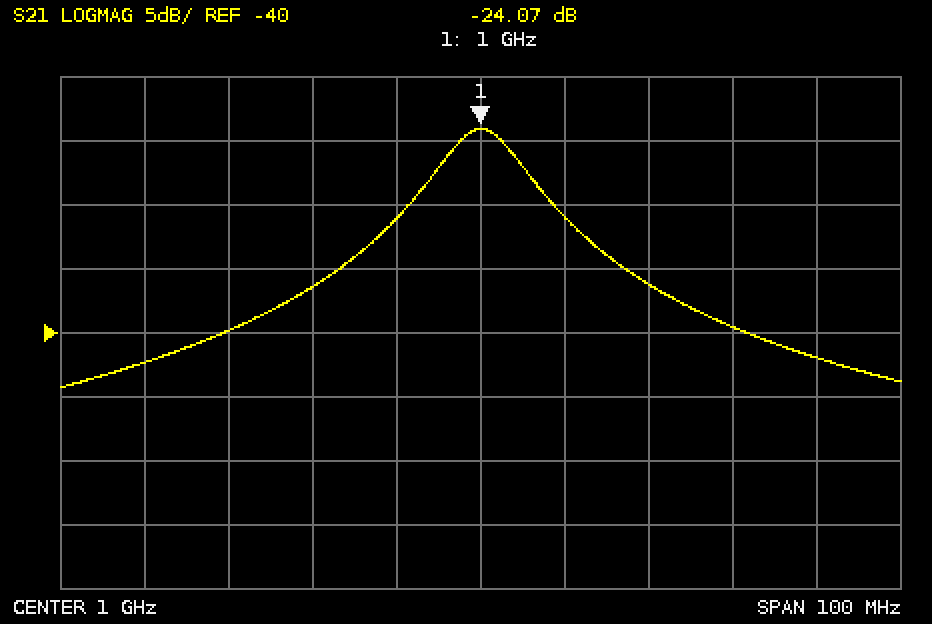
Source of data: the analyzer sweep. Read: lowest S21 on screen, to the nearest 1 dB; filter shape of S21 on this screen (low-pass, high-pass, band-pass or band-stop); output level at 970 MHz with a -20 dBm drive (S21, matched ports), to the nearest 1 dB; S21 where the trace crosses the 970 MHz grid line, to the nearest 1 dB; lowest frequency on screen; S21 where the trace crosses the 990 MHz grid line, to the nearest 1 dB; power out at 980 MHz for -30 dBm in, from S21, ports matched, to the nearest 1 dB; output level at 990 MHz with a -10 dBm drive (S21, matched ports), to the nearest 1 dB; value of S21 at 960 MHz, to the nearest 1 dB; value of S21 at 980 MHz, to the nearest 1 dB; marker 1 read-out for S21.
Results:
-44 dB
band-pass
-60 dBm
-40 dB
950 MHz
-31 dB
-66 dBm
-41 dBm
-42 dB
-36 dB
-24.07 dB
